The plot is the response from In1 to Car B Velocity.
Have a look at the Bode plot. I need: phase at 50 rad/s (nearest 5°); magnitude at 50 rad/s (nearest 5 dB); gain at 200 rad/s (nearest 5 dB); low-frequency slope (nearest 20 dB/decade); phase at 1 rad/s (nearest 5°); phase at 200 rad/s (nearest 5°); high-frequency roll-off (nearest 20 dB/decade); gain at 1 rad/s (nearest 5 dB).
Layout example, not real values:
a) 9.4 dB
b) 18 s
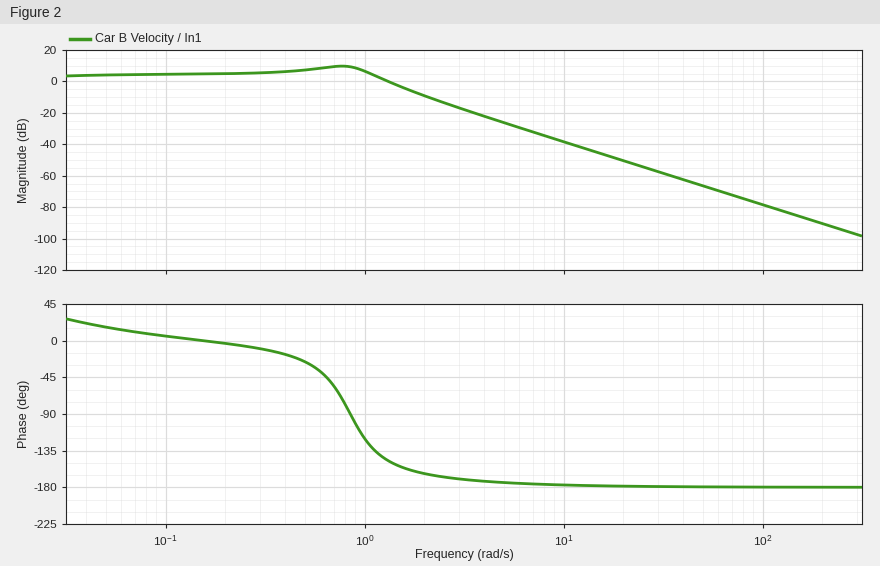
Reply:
a) -180°
b) -65 dB
c) -90 dB
d) 0 dB/decade
e) -120°
f) -180°
g) -40 dB/decade
h) 5 dB
